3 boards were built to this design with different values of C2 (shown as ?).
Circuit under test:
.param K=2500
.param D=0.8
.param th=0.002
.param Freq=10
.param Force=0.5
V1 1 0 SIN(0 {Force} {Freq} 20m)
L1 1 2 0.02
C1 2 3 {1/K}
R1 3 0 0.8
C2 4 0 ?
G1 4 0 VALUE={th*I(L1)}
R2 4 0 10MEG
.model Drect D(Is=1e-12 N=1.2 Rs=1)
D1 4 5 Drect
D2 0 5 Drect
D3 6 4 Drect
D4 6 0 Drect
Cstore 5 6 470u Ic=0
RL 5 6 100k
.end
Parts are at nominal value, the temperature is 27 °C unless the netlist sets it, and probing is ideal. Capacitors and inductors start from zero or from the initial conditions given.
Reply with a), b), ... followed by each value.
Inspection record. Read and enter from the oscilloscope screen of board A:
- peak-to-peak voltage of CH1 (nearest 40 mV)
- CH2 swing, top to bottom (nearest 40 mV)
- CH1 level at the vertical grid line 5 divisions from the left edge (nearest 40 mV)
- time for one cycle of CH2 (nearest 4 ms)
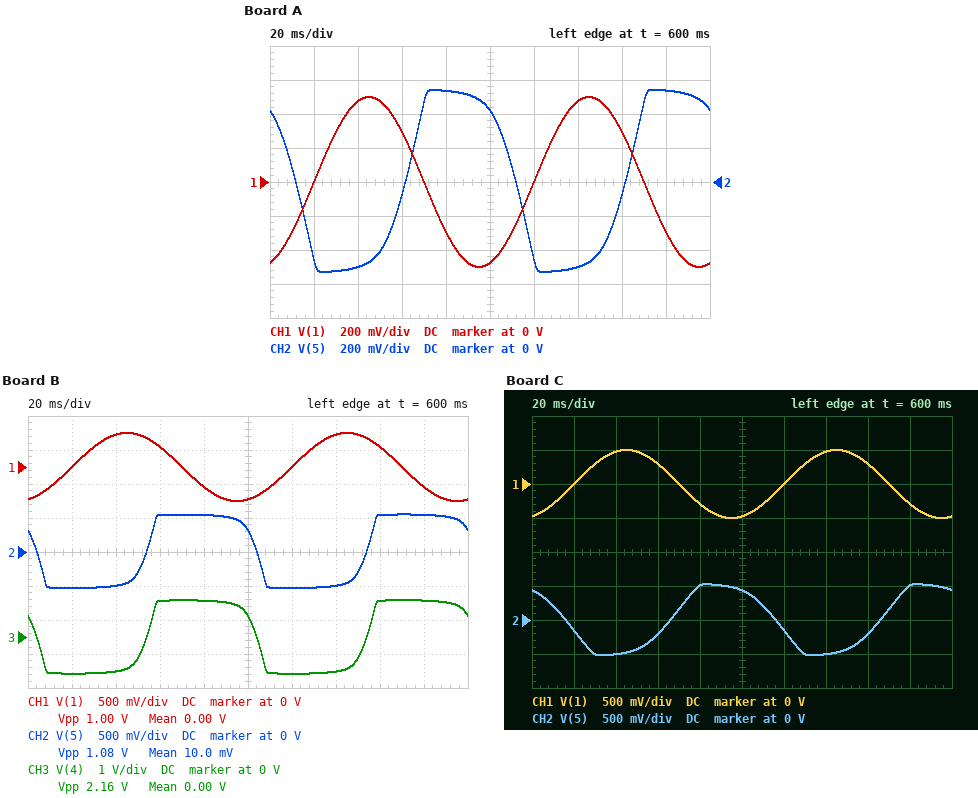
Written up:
a) 1.00 V
b) 1.08 V
c) -480 mV
d) 100 ms
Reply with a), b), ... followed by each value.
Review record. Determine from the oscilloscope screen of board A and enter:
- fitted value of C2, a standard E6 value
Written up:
a) 220 nF
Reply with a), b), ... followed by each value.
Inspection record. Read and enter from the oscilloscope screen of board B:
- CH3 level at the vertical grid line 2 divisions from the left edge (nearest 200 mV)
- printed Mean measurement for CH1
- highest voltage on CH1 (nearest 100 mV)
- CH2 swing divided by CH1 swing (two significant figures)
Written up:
a) -1.0 V
b) 0.00 V
c) 500 mV
d) 1.1
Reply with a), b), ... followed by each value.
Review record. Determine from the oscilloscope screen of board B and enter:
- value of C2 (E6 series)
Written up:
a) 68 nF
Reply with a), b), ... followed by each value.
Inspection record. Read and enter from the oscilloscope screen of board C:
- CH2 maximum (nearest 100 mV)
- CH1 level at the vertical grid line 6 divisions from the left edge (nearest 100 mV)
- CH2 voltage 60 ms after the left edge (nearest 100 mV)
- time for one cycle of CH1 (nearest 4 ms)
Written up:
a) 500 mV
b) 0 V
c) -200 mV
d) 100 ms
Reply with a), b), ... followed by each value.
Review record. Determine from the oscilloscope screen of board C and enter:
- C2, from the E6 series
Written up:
a) 330 nF
